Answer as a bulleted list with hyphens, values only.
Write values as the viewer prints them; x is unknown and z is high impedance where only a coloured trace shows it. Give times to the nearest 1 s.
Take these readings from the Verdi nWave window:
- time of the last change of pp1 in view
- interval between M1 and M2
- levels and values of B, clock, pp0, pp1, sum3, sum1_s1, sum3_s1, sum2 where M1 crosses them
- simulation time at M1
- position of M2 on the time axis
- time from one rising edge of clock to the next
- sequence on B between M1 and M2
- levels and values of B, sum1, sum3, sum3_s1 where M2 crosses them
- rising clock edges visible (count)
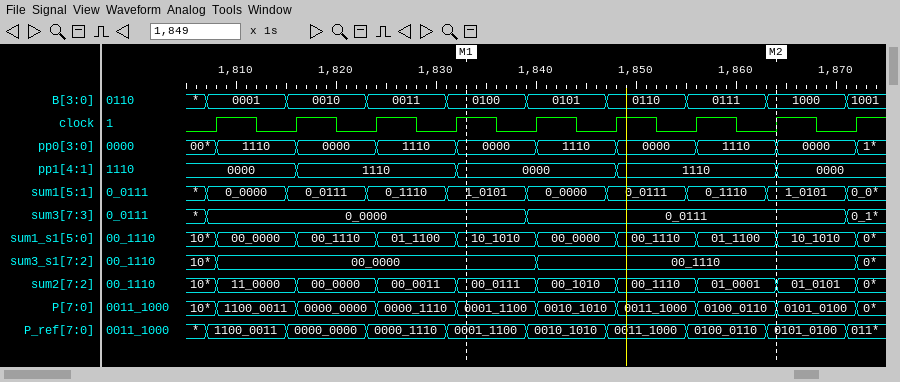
- 1864 s
- 31 s
- B=0100, clock=1, pp0=0000, pp1=0000, sum3=0_0000, sum1_s1=10_1010, sum3_s1=00_0000, sum2=00_0111
- 1833 s
- 1864 s
- 8 s
- 0100, 0101, 0110, 0111, 1000
- B=1000, sum1=1_0101, sum3=0_0111, sum3_s1=00_1110
- 9
